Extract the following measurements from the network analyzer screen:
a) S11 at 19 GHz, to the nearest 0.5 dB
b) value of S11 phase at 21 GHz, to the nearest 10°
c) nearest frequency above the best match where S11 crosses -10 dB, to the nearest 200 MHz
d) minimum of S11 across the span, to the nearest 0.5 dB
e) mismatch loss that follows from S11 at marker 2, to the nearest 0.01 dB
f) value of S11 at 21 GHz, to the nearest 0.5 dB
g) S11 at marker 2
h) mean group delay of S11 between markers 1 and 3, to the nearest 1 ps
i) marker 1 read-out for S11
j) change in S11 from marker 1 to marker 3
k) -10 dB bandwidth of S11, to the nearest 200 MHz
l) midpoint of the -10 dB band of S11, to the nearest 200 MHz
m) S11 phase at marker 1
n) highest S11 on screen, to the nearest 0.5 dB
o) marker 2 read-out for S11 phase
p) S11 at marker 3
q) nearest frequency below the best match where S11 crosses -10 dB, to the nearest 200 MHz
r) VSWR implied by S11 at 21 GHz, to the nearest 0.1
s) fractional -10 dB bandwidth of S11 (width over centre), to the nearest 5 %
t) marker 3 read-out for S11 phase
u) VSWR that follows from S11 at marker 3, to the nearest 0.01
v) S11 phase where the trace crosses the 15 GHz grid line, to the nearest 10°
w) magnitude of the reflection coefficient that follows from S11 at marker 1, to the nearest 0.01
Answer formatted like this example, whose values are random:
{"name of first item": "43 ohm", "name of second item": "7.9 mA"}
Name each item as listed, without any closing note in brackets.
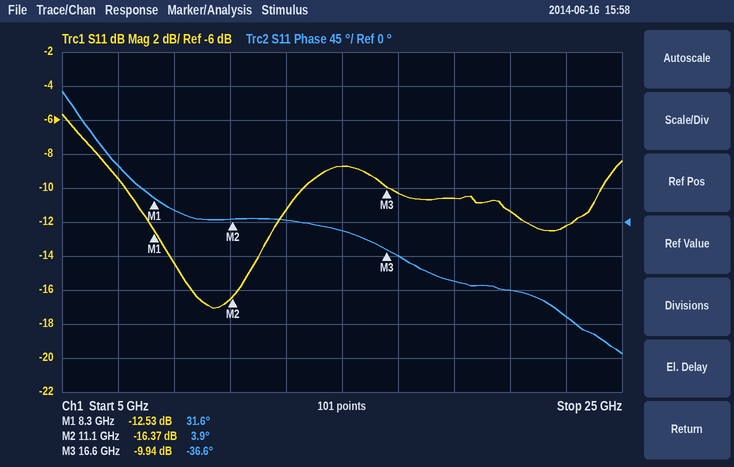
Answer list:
{"S11 at 19 GHz, to the nearest 0.5 dB": "-10.5 dB", "value of S11 phase at 21 GHz, to the nearest 10°": "-90°", "nearest frequency above the best match where S11 crosses -10 dB, to the nearest 200 MHz": "13.6 GHz", "minimum of S11 across the span, to the nearest 0.5 dB": "-17.0 dB", "mismatch loss that follows from S11 at marker 2, to the nearest 0.01 dB": "0.10 dB", "value of S11 at 21 GHz, to the nearest 0.5 dB": "-11.5 dB", "S11 at marker 2": "-16.37 dB", "mean group delay of S11 between markers 1 and 3, to the nearest 1 ps": "23 ps", "marker 1 read-out for S11": "-12.53 dB", "change in S11 from marker 1 to marker 3": "2.59 dB", "-10 dB bandwidth of S11, to the nearest 200 MHz": "6.4 GHz", "midpoint of the -10 dB band of S11, to the nearest 200 MHz": "10.4 GHz", "S11 phase at marker 1": "31.6°", "highest S11 on screen, to the nearest 0.5 dB": "-5.5 dB", "marker 2 read-out for S11 phase": "3.9°", "S11 at marker 3": "-9.94 dB", "nearest frequency below the best match where S11 crosses -10 dB, to the nearest 200 MHz": "7.2 GHz", "VSWR implied by S11 at 21 GHz, to the nearest 0.1": "1.7", "fractional -10 dB bandwidth of S11 (width over centre), to the nearest 5 %": "60 %", "marker 3 read-out for S11 phase": "-36.6°", "VSWR that follows from S11 at marker 3, to the nearest 0.01": "1.93", "S11 phase where the trace crosses the 15 GHz grid line, to the nearest 10°": "-10°", "magnitude of the reflection coefficient that follows from S11 at marker 1, to the nearest 0.01": "0.24"}
